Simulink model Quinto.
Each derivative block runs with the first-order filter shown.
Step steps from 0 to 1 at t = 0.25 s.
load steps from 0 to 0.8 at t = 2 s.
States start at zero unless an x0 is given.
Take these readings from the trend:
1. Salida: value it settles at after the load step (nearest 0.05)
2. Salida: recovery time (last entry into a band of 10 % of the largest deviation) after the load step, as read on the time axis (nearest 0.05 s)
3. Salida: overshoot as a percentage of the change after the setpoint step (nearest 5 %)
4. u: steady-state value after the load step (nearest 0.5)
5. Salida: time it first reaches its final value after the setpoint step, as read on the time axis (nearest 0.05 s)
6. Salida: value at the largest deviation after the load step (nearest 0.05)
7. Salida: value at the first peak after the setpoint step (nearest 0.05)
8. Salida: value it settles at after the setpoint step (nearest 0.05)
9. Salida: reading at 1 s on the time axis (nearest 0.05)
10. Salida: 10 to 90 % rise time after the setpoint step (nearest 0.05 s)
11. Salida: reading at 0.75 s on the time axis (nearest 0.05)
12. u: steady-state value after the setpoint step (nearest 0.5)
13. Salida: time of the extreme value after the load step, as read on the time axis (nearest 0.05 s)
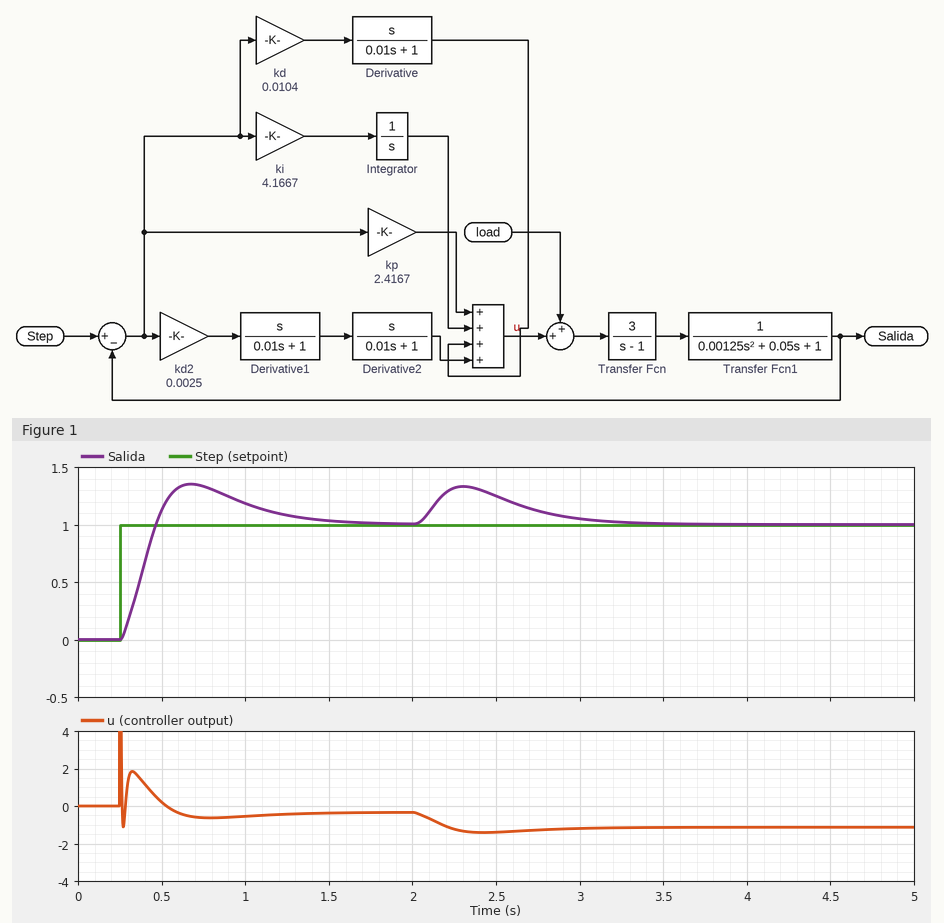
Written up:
1.00
3.10 s
35 %
-1.0
0.45 s
1.35
1.35
1.00
1.20
0.15 s
1.35
-0.5
2.30 s
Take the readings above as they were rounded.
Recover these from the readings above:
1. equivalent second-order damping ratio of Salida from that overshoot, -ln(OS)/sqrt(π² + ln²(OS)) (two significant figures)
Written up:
0.32
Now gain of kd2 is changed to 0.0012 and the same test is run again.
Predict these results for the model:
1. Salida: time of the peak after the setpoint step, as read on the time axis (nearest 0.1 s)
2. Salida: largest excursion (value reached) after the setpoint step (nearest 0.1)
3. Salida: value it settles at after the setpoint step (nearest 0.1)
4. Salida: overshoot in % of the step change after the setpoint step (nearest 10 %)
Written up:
0.7 s
1.3
1.0
30 %
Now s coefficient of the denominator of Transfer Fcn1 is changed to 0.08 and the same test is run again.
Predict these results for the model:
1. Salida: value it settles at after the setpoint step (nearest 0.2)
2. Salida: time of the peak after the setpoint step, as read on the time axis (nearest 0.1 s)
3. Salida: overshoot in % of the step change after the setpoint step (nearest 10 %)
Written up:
1.0
0.7 s
50 %
